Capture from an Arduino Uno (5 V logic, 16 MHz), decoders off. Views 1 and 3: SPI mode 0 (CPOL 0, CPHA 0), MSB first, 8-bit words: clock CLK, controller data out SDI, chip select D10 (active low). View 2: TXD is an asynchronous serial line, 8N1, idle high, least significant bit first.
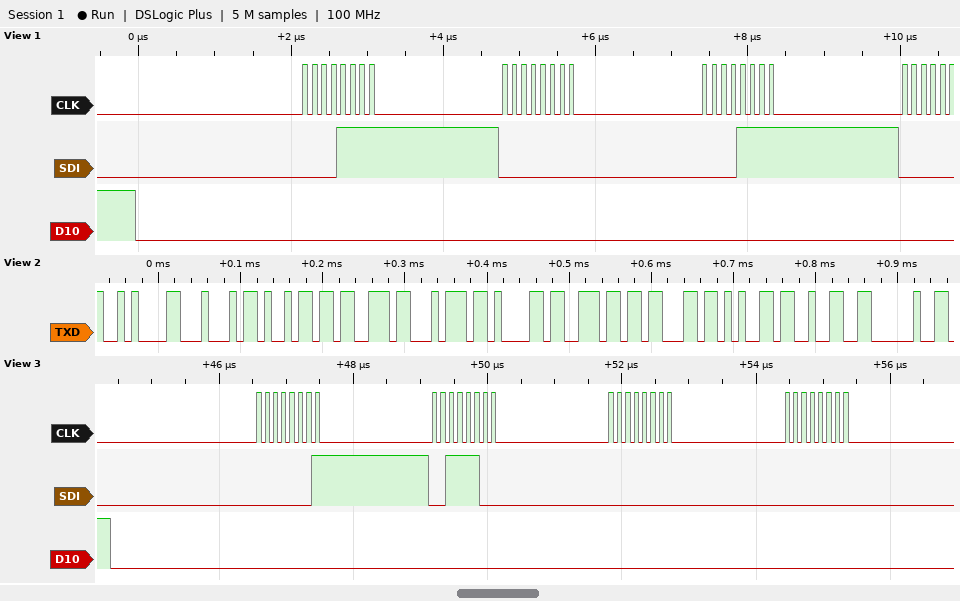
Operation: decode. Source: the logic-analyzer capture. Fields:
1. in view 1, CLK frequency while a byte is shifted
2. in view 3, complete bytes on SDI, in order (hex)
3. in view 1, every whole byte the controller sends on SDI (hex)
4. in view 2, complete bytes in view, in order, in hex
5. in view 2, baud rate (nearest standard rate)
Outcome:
8 MHz
01 3C 00 00
0F 00 0F
0A 44 69 73 74 61 6E 63 65 32 20
115200 baud
